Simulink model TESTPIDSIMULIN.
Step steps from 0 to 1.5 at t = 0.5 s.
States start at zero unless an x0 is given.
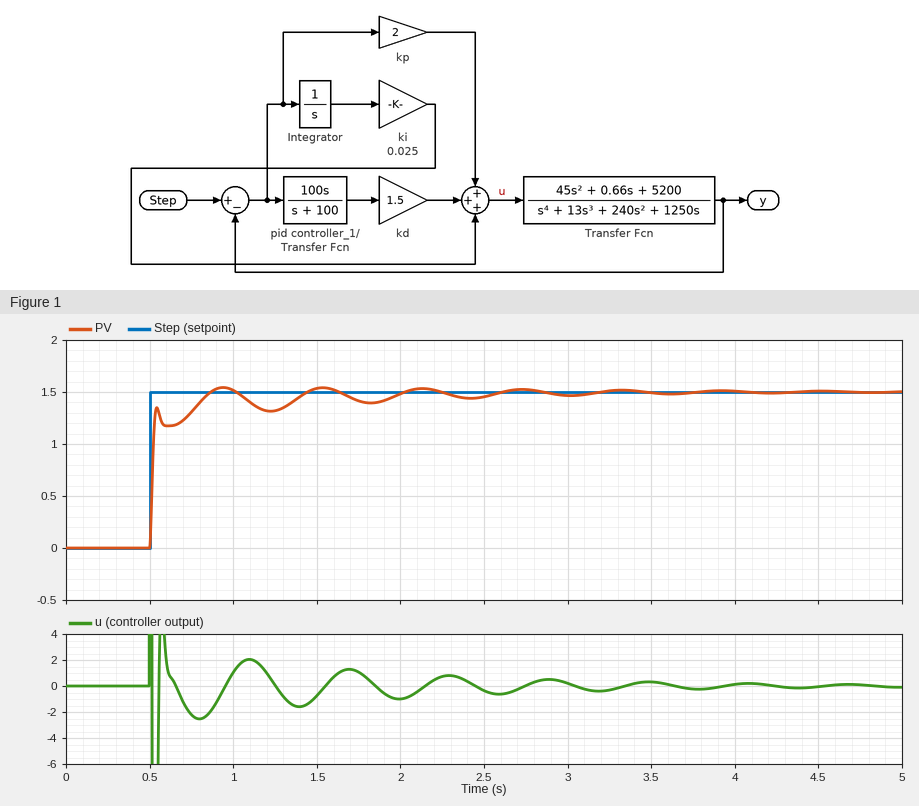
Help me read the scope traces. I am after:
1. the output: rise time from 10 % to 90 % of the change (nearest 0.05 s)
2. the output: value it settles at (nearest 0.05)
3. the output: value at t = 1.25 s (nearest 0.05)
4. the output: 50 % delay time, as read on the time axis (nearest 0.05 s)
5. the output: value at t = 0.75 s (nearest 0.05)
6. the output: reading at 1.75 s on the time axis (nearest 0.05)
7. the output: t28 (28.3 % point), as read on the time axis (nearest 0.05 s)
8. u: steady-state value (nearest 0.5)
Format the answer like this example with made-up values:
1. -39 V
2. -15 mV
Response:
1. 0.25 s
2. 1.50
3. 1.30
4. 0.50 s
5. 1.30
6. 1.40
7. 0.50 s
8. 0.0
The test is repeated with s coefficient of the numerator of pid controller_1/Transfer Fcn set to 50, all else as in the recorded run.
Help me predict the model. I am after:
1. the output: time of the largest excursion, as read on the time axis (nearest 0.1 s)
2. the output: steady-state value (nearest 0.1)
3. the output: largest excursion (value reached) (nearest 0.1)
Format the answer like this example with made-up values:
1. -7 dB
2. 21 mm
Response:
1. 1.0 s
2. 1.5
3. 1.6
